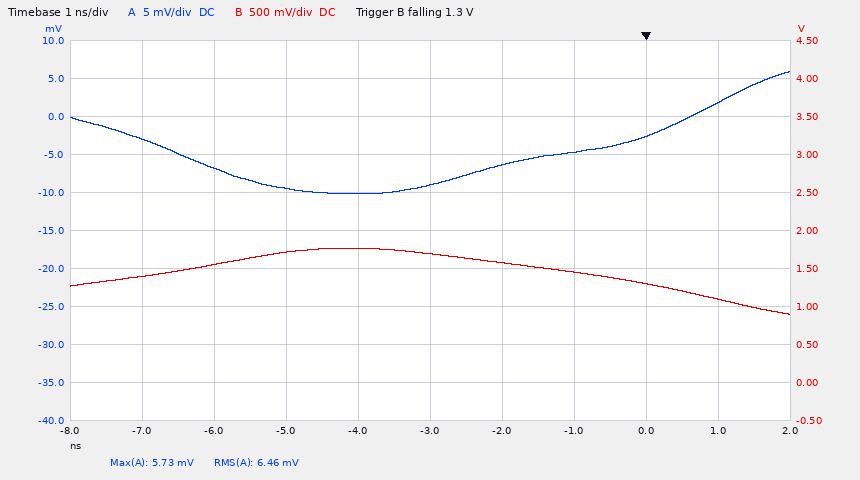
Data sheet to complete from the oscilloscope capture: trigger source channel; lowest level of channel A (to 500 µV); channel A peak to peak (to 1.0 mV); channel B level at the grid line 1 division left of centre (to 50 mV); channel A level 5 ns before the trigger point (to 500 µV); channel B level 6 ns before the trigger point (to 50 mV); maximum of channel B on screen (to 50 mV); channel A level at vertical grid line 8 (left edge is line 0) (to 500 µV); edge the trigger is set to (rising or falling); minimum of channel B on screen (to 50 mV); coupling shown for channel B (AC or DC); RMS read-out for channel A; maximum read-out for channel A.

channel B
-10.0 mV
16.0 mV
1.75 V
-9.5 mV
1.55 V
1.75 V
-2.5 mV
falling
900 mV
DC
6.46 mV
5.73 mV
